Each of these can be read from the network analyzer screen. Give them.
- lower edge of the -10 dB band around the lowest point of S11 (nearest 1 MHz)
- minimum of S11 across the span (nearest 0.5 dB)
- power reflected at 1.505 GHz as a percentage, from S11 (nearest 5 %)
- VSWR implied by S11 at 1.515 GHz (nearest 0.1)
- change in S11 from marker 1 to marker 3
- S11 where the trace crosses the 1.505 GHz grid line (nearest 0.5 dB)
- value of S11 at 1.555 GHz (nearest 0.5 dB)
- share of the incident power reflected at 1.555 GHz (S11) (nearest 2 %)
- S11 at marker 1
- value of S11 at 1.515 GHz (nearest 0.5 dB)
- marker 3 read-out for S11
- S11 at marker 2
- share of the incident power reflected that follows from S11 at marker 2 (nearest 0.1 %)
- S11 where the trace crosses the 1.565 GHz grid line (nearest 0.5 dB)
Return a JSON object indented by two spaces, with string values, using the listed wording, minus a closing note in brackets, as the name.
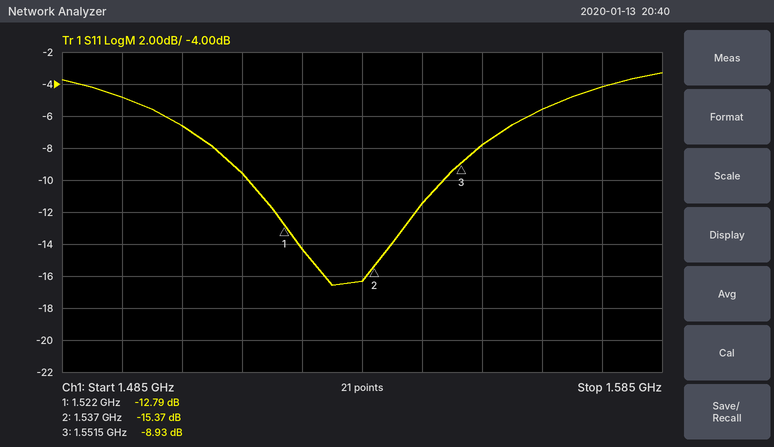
{
  "lower edge of the -10 dB band around the lowest point of S11": "1.516 GHz",
  "minimum of S11 across the span": "-16.5 dB",
  "power reflected at 1.505 GHz as a percentage, from S11": "20 %",
  "VSWR implied by S11 at 1.515 GHz": "2.0",
  "change in S11 from marker 1 to marker 3": "3.86 dB",
  "S11 where the trace crosses the 1.505 GHz grid line": "-6.5 dB",
  "value of S11 at 1.555 GHz": "-8.0 dB",
  "share of the incident power reflected at 1.555 GHz (S11)": "16 %",
  "S11 at marker 1": "-12.79 dB",
  "value of S11 at 1.515 GHz": "-9.5 dB",
  "marker 3 read-out for S11": "-8.93 dB",
  "S11 at marker 2": "-15.37 dB",
  "share of the incident power reflected that follows from S11 at marker 2": "2.9 %",
  "S11 where the trace crosses the 1.565 GHz grid line": "-5.5 dB"
}
